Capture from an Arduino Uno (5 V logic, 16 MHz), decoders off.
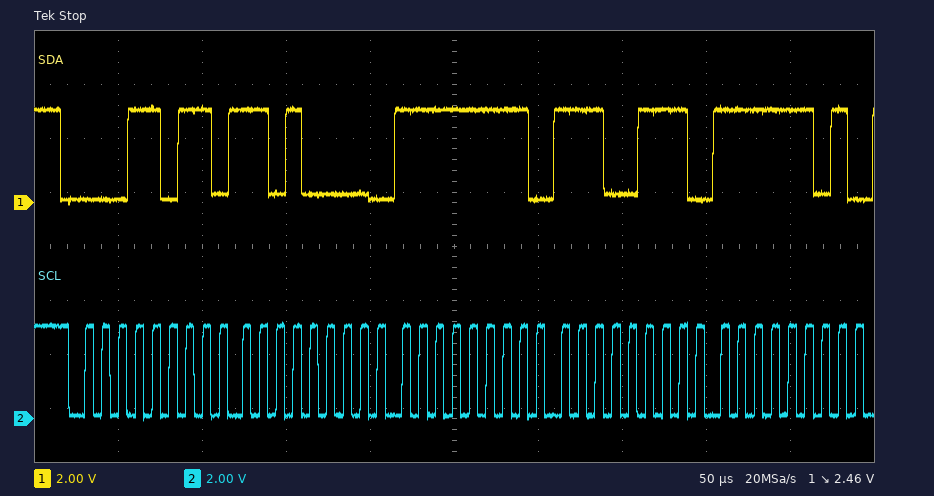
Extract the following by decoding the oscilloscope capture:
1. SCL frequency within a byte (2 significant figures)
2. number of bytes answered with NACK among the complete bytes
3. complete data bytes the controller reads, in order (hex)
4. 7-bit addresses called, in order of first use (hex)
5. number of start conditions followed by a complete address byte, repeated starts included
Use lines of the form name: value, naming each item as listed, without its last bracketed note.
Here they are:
SCL frequency within a byte: 100 kHz
number of bytes answered with NACK among the complete bytes: 0
complete data bytes the controller reads, in order: D0 FF E7 FD
7-bit addresses called, in order of first use: 0x0D
number of start conditions followed by a complete address byte, repeated starts included: 1
